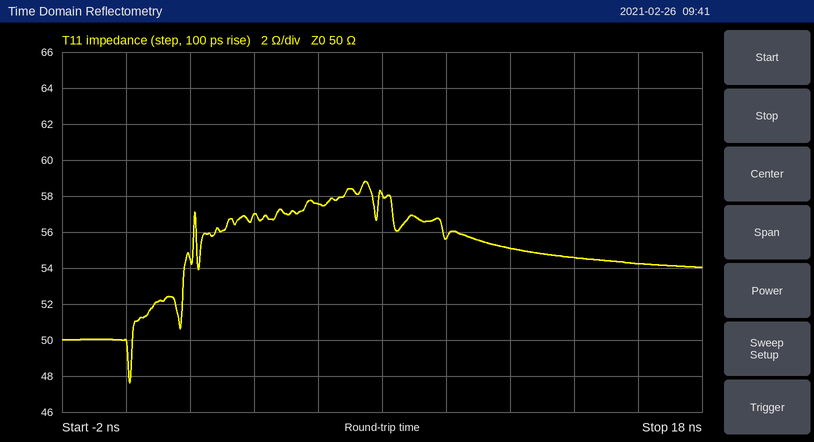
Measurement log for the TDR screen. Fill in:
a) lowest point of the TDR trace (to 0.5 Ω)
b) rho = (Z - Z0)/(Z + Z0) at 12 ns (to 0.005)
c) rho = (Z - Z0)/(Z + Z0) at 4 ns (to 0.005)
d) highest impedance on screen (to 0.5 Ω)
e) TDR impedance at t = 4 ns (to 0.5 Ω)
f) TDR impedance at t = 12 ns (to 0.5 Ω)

47.5 Ω
+0.050
+0.065
59.0 Ω
57.0 Ω
55.0 Ω
